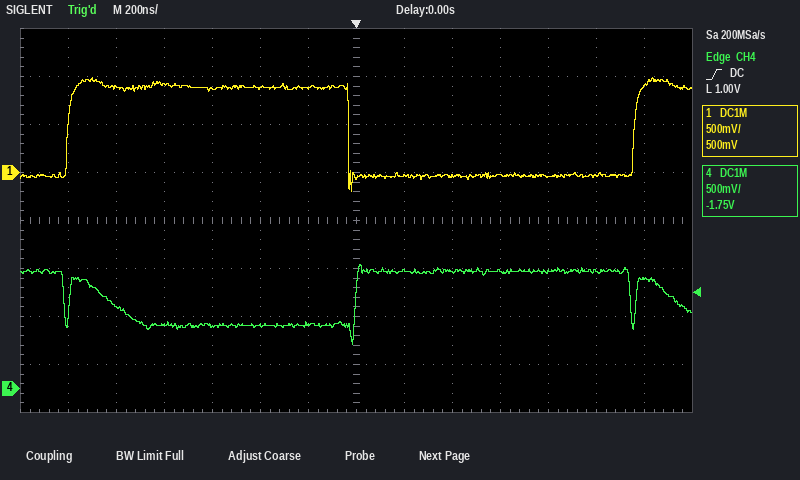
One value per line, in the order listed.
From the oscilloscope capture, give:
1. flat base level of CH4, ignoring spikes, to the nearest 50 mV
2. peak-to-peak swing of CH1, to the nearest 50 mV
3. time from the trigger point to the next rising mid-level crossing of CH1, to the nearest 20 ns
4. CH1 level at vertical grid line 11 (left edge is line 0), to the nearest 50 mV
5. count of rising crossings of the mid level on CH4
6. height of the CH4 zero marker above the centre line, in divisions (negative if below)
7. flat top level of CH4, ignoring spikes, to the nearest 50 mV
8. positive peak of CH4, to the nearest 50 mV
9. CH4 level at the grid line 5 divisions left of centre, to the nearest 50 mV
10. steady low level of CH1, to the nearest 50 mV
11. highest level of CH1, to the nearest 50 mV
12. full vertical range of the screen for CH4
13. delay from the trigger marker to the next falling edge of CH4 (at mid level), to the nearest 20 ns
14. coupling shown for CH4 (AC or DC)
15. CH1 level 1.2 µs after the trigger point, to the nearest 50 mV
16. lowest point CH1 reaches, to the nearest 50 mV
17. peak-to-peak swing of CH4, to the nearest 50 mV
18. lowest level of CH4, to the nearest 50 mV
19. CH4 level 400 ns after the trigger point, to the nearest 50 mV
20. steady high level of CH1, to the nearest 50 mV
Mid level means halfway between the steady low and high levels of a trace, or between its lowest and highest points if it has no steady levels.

650 mV
1.20 V
1.16 µs
-50 mV
3
-3.5 div
1.20 V
1.30 V
850 mV
-50 mV
1.00 V
4 V
1.14 µs
DC
900 mV
-200 mV
850 mV
450 mV
1.20 V
900 mV
